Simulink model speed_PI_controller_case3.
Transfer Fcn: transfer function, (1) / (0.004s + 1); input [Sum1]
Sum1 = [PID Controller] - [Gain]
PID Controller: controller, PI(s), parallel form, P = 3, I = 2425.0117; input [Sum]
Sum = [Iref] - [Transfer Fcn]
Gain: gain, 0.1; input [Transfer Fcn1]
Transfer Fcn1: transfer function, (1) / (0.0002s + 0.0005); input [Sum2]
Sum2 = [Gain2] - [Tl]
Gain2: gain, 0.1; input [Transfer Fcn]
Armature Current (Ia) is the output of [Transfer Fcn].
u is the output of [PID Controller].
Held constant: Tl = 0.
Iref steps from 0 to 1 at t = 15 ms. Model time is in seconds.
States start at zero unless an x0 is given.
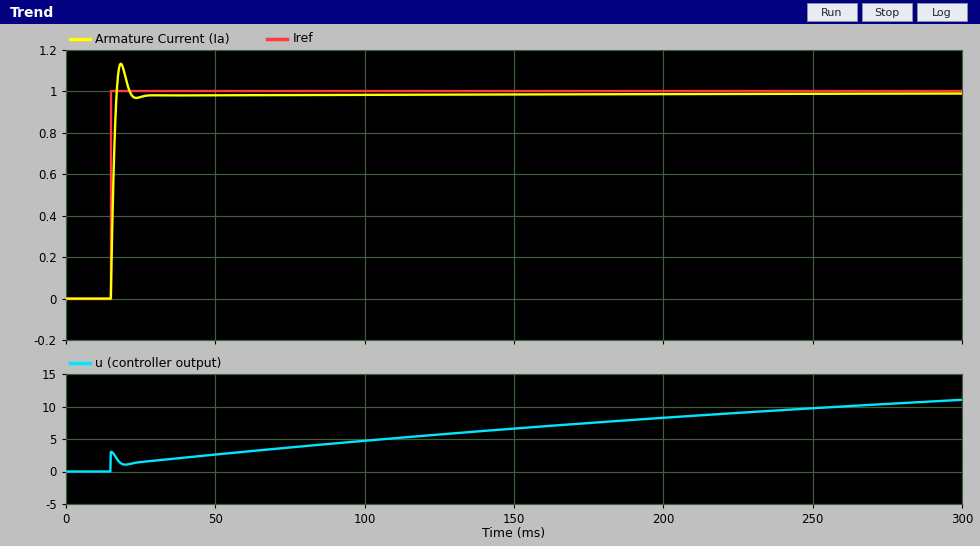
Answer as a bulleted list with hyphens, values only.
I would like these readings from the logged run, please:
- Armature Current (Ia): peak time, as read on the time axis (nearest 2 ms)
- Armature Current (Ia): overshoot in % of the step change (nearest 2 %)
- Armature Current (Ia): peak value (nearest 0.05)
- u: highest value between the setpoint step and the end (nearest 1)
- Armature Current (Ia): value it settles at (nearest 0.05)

- 18 ms
- 14 %
- 1.15
- 11
- 1.00
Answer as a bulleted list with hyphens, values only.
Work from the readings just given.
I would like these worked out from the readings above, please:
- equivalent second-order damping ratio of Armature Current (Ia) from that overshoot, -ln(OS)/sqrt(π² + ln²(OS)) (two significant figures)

- 0.53
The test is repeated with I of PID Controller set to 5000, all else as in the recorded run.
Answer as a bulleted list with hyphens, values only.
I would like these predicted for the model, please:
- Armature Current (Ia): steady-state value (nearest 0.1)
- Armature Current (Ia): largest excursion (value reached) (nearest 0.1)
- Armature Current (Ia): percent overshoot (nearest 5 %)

- 1.0
- 1.3
- 25 %
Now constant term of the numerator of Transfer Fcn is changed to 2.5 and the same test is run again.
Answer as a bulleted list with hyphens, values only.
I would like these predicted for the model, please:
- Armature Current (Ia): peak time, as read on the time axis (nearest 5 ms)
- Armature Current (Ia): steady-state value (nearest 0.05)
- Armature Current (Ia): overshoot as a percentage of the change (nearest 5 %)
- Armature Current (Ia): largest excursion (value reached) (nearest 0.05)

- 15 ms
- 1.00
- 10 %
- 1.10
